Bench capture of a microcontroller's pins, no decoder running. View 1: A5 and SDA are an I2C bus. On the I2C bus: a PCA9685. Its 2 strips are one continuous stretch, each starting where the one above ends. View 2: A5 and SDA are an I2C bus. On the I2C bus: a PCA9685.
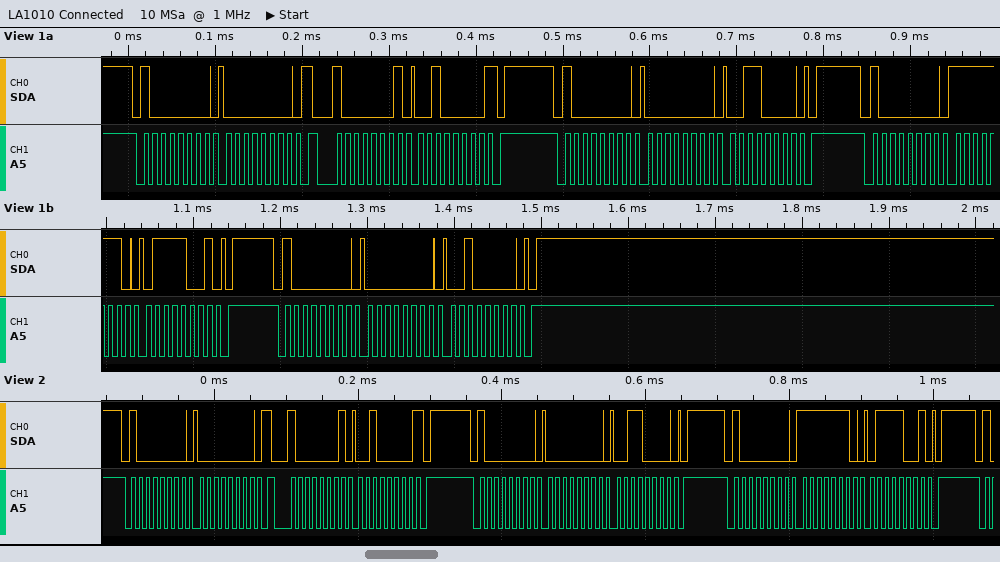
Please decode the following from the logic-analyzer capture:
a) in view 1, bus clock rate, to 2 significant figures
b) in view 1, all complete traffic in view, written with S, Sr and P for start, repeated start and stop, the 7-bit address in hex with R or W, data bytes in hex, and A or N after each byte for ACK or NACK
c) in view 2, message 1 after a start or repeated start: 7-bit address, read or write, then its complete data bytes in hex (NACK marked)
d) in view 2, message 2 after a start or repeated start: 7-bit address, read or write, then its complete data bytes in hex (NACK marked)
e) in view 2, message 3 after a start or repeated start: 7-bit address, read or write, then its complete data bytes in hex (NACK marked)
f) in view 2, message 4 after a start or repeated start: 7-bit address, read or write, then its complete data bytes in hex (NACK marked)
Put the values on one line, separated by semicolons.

100 kHz; S 40W A 00 A Sr 40R A 20 N P S 40W A 00 A 30 A P S 40W A FE A 79 A P S 40W A 00 A 20 A P; 0x40 write: 00; 0x40 read: 20 NACK; 0x40 write: 00 30; 0x40 write: FE 79
